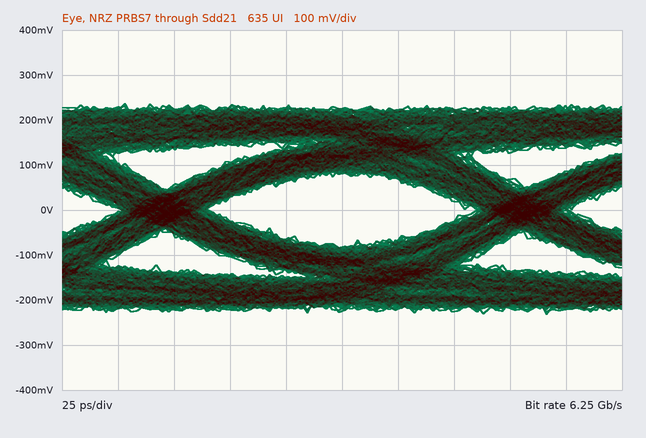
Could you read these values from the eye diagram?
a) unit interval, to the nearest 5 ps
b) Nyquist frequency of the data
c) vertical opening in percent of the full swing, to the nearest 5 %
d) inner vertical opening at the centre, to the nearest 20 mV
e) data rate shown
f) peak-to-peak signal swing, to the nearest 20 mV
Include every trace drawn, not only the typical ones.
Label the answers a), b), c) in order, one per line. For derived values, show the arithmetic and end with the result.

a) 160 ps
b) 3.125 GHz
c) 160 mV / 460 mV ≈ 35 %
d) 160 mV
e) 6.25 Gb/s
f) 460 mV
